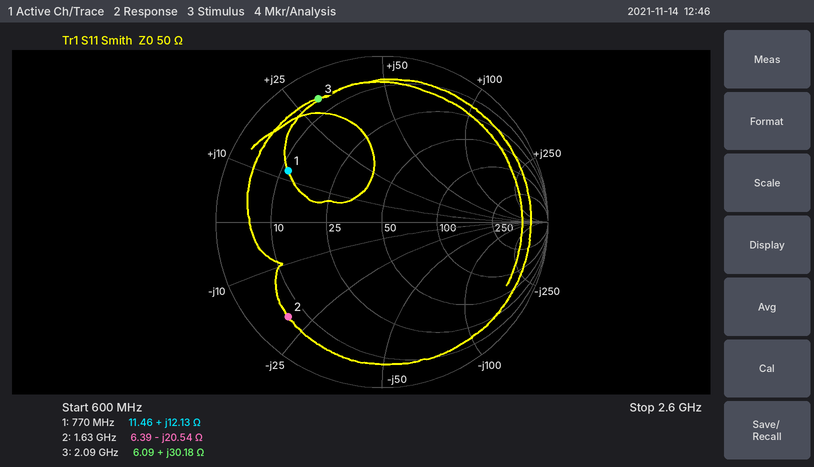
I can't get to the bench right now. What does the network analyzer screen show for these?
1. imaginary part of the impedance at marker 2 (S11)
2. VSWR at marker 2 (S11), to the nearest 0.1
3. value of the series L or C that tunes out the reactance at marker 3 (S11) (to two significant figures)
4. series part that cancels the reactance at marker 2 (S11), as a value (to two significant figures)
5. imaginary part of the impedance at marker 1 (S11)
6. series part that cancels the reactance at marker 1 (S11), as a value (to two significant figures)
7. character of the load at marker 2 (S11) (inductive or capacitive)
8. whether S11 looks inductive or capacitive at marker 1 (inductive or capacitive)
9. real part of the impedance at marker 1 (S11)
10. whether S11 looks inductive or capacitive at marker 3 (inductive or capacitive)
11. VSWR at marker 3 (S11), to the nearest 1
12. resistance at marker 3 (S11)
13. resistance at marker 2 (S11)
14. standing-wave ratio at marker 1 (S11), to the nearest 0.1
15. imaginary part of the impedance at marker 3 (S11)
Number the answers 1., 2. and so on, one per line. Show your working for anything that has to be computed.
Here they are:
1. -20.54 Ω
2. 9.2
3. C = 1/(2π × 2.09 GHz × 30.18 Ω) ≈ 2.5 pF
4. L = 20.54 Ω/(2π × 1.63 GHz) ≈ 2.0 nH
5. +12.13 Ω
6. C = 1/(2π × 770 MHz × 12.13 Ω) ≈ 17 pF
7. capacitive
8. inductive
9. 11.46 Ω
10. inductive
11. 11
12. 6.09 Ω
13. 6.39 Ω
14. 4.6
15. +30.18 Ω
